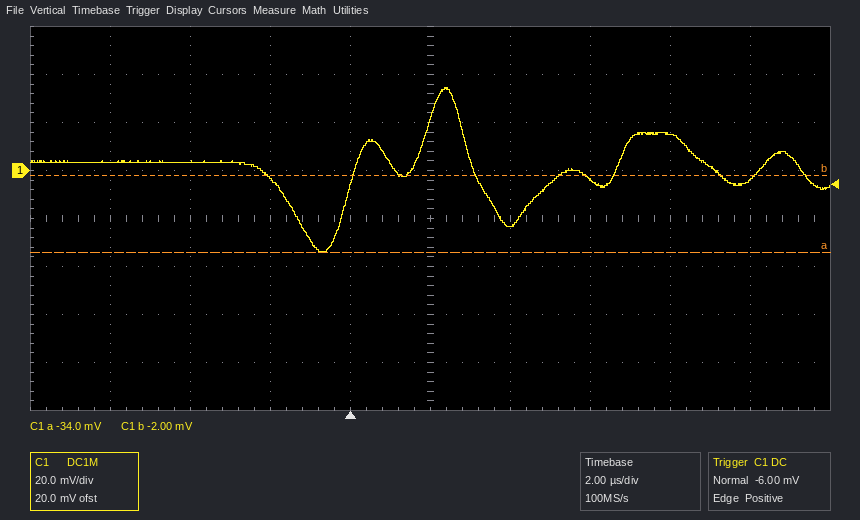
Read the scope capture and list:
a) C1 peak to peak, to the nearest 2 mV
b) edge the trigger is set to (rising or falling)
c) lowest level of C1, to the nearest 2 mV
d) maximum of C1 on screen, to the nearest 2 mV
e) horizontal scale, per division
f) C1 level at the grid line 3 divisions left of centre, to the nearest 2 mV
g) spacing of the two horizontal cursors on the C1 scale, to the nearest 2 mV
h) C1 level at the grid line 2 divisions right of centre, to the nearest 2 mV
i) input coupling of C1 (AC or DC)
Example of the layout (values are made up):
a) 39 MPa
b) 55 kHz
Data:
a) 68 mV
b) rising
c) -34 mV
d) 34 mV
e) 2 µs
f) 4 mV
g) 32 mV
h) -4 mV
i) DC
